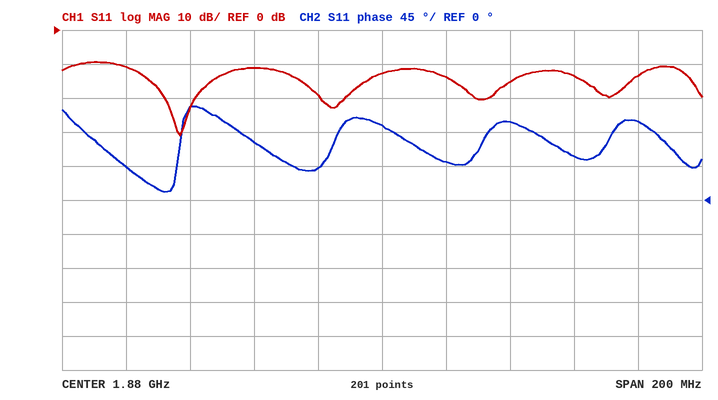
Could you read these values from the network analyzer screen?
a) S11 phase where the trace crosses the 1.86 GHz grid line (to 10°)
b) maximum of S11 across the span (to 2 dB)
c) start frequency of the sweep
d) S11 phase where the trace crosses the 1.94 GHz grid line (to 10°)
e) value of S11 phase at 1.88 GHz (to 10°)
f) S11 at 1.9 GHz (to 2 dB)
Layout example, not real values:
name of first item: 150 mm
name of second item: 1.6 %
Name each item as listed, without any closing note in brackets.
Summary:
S11 phase where the trace crosses the 1.86 GHz grid line: 40°
maximum of S11 across the span: -10 dB
start frequency of the sweep: 1.78 GHz
S11 phase where the trace crosses the 1.94 GHz grid line: 60°
value of S11 phase at 1.88 GHz: 100°
S11 at 1.9 GHz: -14 dB
